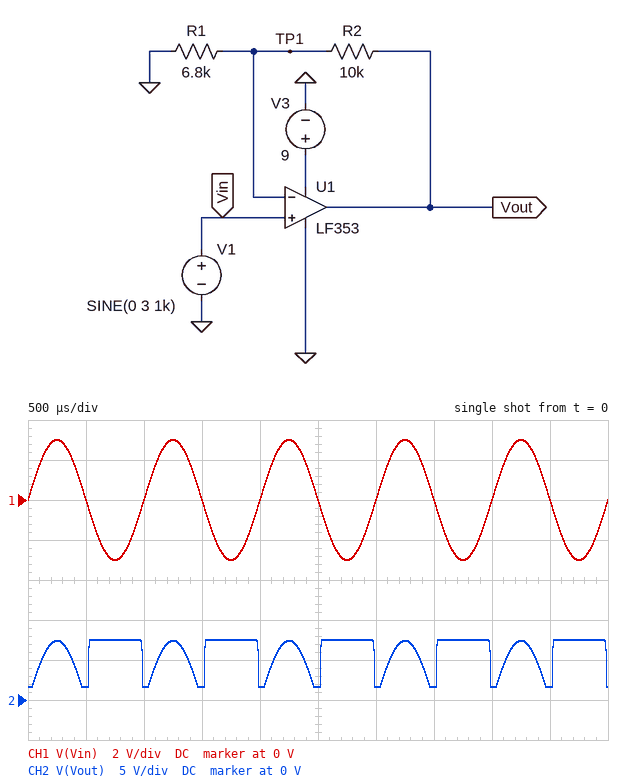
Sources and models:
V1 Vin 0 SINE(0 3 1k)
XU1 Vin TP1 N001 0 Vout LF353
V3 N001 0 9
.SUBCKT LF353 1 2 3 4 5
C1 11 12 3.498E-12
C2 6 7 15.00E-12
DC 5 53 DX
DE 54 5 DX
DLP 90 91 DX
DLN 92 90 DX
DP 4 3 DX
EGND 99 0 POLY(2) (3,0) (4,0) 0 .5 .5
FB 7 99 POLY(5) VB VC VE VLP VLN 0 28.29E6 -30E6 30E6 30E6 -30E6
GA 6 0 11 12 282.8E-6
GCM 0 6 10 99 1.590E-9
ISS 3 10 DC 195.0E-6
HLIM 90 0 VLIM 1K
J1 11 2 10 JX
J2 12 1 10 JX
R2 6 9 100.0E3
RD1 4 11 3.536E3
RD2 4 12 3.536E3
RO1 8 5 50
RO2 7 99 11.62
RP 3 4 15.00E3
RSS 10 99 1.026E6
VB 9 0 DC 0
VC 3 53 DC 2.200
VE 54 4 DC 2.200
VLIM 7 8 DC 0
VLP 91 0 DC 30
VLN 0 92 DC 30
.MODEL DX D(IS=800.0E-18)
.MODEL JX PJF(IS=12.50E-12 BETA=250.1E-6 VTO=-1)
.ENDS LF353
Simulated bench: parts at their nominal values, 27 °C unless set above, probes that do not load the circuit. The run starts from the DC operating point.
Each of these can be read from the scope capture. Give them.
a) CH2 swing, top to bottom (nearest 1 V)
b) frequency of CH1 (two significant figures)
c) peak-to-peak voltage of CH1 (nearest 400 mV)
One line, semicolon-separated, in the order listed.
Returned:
6 V; 1.0 kHz; 6.0 V
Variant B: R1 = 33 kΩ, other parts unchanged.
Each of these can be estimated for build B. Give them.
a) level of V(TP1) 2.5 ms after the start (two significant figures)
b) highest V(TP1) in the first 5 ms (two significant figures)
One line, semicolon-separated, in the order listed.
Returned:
1.2 V; 5.8 V
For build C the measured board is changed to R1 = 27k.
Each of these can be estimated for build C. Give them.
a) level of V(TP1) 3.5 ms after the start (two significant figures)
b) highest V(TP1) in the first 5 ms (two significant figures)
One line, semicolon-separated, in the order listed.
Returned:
1.1 V; 5.5 V
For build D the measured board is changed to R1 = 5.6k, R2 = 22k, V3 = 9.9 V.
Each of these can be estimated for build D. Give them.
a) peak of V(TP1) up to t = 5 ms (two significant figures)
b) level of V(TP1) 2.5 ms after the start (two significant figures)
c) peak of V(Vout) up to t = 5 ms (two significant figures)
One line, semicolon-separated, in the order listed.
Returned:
1.7 V; 330 mV; 8.4 V
